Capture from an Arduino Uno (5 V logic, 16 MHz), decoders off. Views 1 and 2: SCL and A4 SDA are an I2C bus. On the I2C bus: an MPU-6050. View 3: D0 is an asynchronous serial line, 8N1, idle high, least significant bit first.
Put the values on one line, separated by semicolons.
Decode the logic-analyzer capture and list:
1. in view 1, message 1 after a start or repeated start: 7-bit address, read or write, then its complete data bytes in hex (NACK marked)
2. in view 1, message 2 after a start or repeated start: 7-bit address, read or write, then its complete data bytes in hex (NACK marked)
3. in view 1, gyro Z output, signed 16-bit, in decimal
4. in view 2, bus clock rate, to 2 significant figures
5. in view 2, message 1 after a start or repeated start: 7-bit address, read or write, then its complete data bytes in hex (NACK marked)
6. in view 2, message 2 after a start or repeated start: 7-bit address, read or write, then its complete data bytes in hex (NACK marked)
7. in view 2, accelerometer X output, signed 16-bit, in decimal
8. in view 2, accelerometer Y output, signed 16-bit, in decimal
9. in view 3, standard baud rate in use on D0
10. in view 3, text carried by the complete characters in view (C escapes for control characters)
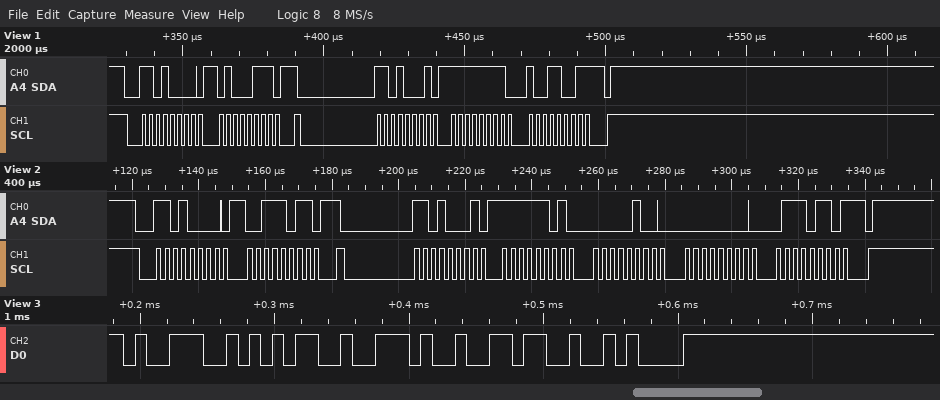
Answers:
0x68 write: 47; 0x68 read: FF 99 NACK; -103; 400 kHz; 0x68 write: 3B; 0x68 read: FD 04 00 76 NACK; -764; 118; 115200 baud; "95.6\n"
